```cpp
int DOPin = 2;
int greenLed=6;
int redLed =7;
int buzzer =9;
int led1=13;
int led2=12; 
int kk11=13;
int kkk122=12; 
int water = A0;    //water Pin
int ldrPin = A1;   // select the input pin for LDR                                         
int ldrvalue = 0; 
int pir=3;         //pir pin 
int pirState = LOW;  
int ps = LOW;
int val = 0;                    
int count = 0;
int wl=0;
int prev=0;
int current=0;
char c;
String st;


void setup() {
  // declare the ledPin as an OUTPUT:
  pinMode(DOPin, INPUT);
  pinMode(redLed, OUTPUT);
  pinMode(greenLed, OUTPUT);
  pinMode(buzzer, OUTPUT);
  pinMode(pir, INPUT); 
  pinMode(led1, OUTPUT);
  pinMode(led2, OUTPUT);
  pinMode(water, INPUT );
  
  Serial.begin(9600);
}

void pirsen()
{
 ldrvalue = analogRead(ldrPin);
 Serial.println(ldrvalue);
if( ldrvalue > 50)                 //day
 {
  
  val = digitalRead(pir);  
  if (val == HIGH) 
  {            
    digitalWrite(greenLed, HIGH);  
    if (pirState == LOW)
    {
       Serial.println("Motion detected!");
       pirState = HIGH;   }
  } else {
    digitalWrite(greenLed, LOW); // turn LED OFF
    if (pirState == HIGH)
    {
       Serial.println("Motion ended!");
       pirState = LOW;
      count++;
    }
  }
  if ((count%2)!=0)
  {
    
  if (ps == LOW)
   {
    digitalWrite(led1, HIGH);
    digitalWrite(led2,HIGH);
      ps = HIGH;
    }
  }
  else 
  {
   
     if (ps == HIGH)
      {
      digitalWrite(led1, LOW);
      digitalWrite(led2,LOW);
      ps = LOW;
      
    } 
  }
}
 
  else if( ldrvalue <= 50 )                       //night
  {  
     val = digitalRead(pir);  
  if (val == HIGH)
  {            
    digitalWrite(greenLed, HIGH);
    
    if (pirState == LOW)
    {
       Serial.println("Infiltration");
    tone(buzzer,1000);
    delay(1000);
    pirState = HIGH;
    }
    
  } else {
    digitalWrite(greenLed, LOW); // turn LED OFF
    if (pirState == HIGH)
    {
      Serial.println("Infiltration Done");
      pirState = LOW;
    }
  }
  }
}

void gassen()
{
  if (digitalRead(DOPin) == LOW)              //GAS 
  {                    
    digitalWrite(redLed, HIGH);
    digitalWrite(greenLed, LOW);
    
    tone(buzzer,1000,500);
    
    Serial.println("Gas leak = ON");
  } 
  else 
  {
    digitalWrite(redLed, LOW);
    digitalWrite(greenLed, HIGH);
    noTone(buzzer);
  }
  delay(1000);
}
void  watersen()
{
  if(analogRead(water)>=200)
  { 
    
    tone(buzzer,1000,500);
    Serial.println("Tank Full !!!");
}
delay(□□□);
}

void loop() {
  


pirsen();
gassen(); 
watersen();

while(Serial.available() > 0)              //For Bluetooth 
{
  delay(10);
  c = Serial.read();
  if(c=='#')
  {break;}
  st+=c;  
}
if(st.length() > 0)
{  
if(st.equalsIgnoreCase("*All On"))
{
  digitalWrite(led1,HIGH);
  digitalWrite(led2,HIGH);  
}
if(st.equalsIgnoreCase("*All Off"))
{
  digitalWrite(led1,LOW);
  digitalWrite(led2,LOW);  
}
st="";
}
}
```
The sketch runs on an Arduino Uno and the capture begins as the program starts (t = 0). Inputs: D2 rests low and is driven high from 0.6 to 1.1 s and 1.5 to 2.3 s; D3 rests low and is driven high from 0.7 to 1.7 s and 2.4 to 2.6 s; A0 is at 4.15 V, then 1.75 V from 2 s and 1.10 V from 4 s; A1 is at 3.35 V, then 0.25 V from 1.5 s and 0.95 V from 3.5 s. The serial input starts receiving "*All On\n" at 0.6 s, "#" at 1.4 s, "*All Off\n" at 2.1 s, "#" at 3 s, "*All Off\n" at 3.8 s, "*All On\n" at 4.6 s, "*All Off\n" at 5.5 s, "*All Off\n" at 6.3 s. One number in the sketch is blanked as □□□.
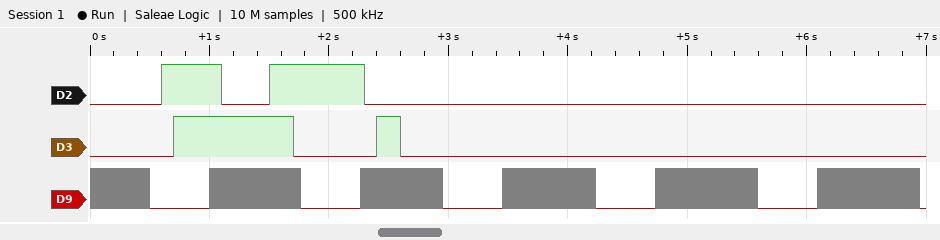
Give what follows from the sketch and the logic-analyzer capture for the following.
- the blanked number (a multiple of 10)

180
